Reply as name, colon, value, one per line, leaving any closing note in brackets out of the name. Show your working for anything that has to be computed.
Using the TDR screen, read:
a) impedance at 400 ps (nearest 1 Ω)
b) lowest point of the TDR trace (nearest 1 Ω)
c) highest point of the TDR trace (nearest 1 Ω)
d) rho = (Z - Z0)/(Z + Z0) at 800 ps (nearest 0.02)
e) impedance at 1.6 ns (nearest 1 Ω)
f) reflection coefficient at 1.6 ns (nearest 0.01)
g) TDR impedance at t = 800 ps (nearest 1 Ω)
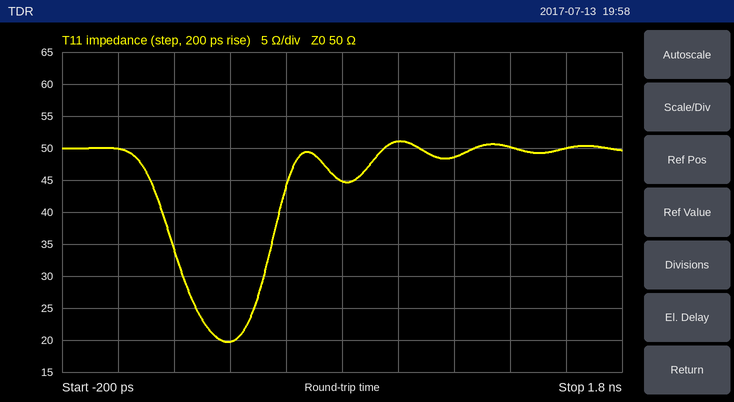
impedance at 400 ps: 20 Ω
lowest point of the TDR trace: 20 Ω
highest point of the TDR trace: 51 Ω
rho = (Z - Z0)/(Z + Z0) at 800 ps: (45 − 50)/(45 + 50) ≈ -0.0526, so -0.06 to the nearest 0.02
impedance at 1.6 ns: 50 Ω
reflection coefficient at 1.6 ns: (50 − 50)/(50 + 50) ≈ 0.00
TDR impedance at t = 800 ps: 45 Ω
